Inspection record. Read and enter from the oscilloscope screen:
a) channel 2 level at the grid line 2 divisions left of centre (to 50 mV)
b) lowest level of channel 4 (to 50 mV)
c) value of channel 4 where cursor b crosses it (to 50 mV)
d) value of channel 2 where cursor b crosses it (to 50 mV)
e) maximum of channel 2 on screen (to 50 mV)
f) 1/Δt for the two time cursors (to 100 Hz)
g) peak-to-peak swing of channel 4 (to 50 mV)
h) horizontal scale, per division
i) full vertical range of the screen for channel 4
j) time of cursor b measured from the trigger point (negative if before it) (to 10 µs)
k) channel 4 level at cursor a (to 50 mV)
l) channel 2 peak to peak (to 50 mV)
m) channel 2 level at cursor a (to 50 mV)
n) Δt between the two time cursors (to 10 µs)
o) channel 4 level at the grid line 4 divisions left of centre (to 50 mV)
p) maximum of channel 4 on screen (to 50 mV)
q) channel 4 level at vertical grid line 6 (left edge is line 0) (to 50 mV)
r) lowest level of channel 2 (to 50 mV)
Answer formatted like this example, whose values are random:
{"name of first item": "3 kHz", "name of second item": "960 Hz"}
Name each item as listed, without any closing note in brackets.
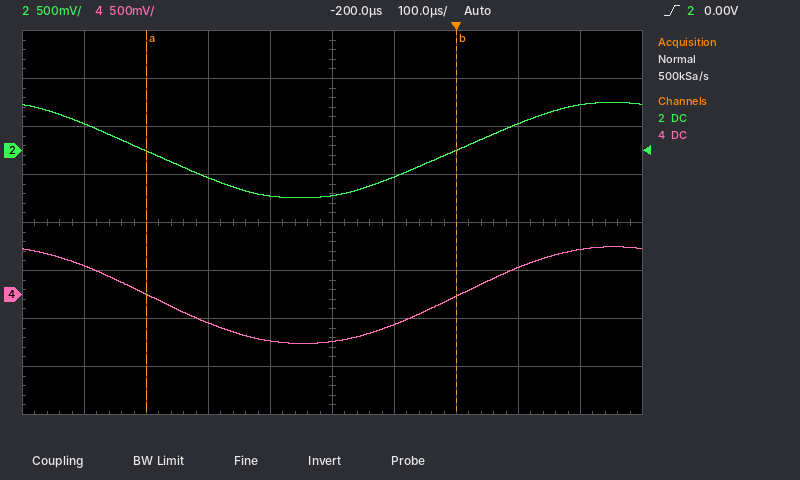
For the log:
{"channel 2 level at the grid line 2 divisions left of centre": "-300 mV", "lowest level of channel 4": "-500 mV", "value of channel 4 where cursor b crosses it": "0 mV", "value of channel 2 where cursor b crosses it": "0 mV", "maximum of channel 2 on screen": "500 mV", "1/Δt for the two time cursors": "2.0 kHz", "peak-to-peak swing of channel 4": "1.00 V", "horizontal scale, per division": "100 µs", "full vertical range of the screen for channel 4": "4 V", "time of cursor b measured from the trigger point (negative if before it)": "0 µs", "channel 4 level at cursor a": "0 mV", "channel 2 peak to peak": "1.00 V", "channel 2 level at cursor a": "0 mV", "Δt between the two time cursors": "500 µs", "channel 4 level at the grid line 4 divisions left of centre": "300 mV", "maximum of channel 4 on screen": "500 mV", "channel 4 level at vertical grid line 6 (left edge is line 0)": "-300 mV", "lowest level of channel 2": "-500 mV"}
